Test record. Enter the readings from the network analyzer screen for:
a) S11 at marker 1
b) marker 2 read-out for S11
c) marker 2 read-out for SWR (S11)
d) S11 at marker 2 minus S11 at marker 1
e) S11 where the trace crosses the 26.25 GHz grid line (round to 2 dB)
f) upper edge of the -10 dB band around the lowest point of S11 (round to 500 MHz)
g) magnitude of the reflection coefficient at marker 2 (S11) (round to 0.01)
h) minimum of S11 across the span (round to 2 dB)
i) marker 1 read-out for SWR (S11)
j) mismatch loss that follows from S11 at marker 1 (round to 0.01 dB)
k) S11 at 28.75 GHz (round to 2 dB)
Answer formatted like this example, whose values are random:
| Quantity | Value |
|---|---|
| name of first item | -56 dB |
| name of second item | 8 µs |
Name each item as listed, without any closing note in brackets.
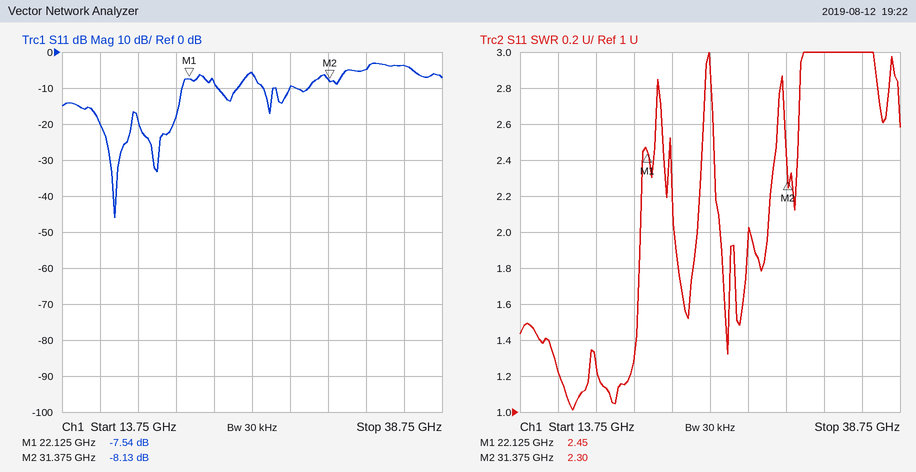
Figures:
| Quantity | Value |
|---|---|
| S11 at marker 1 | -7.54 dB |
| marker 2 read-out for S11 | -8.13 dB |
| marker 2 read-out for SWR | 2.30 |
| S11 at marker 2 minus S11 at marker 1 | -0.59 dB |
| S11 where the trace crosses the 26.25 GHz grid line | -6 dB |
| upper edge of the -10 dB band around the lowest point of S11 | 21.5 GHz |
| magnitude of the reflection coefficient at marker 2 (S11) | 0.39 |
| minimum of S11 across the span | -46 dB |
| marker 1 read-out for SWR | 2.45 |
| mismatch loss that follows from S11 at marker 1 | 0.84 dB |
| S11 at 28.75 GHz | -10 dB |
